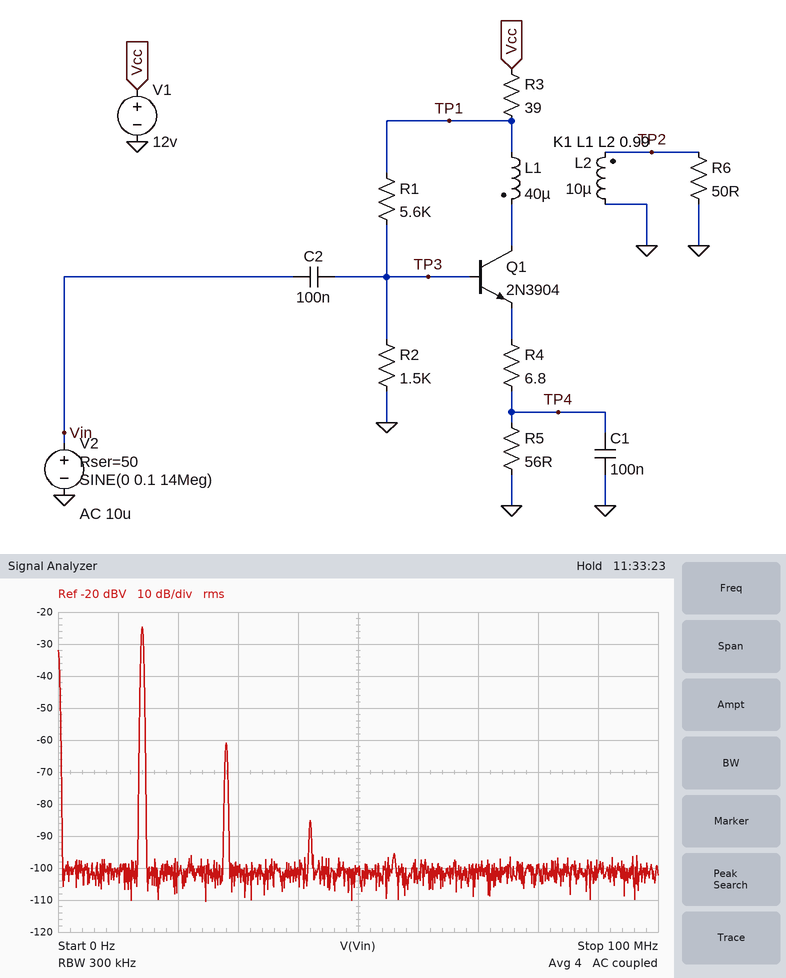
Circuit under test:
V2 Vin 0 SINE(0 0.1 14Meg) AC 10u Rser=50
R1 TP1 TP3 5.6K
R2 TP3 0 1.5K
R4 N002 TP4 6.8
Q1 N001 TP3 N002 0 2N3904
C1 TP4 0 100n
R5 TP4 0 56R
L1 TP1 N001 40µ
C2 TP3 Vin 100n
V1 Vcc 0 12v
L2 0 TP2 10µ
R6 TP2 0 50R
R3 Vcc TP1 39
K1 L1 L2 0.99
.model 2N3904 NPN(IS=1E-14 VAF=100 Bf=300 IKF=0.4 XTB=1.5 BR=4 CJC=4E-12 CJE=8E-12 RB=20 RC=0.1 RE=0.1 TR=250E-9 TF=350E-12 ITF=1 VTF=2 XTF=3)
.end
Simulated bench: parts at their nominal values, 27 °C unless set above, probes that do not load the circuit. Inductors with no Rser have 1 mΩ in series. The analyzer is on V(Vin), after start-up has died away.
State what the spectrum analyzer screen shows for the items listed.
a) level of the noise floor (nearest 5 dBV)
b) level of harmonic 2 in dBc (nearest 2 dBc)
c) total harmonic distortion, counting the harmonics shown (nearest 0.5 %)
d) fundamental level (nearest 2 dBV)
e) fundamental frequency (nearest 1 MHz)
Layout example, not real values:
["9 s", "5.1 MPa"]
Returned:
["-100 dBV", "-36 dBc", "1.5 %", "-24 dBV", "14 MHz"]
